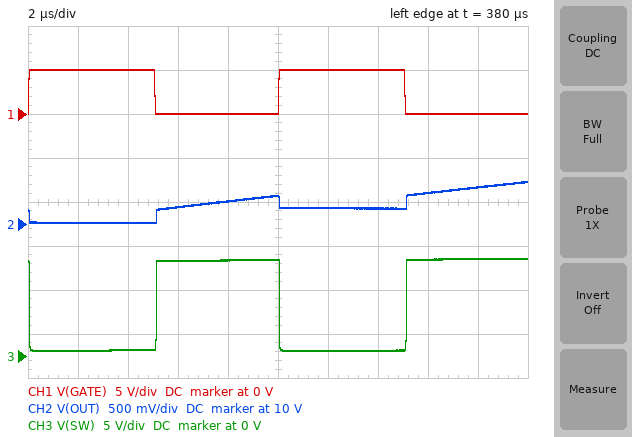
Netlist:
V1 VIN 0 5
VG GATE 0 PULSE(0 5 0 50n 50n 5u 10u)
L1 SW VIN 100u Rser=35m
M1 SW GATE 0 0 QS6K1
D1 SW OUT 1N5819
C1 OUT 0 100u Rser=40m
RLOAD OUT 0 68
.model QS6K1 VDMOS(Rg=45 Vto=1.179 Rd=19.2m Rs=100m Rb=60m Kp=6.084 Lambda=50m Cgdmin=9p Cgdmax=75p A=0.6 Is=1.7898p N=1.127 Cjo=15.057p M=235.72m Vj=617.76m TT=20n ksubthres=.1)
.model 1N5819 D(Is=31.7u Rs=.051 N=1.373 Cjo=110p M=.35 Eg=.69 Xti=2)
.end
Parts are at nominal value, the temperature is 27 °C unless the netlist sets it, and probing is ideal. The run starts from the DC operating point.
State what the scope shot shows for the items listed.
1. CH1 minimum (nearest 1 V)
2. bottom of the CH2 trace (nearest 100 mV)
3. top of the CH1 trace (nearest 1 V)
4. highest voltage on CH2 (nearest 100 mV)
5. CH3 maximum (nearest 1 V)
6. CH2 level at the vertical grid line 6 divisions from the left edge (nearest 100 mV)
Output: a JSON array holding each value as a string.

["0 V", "10.0 V", "5 V", "10.5 V", "11 V", "10.2 V"]
